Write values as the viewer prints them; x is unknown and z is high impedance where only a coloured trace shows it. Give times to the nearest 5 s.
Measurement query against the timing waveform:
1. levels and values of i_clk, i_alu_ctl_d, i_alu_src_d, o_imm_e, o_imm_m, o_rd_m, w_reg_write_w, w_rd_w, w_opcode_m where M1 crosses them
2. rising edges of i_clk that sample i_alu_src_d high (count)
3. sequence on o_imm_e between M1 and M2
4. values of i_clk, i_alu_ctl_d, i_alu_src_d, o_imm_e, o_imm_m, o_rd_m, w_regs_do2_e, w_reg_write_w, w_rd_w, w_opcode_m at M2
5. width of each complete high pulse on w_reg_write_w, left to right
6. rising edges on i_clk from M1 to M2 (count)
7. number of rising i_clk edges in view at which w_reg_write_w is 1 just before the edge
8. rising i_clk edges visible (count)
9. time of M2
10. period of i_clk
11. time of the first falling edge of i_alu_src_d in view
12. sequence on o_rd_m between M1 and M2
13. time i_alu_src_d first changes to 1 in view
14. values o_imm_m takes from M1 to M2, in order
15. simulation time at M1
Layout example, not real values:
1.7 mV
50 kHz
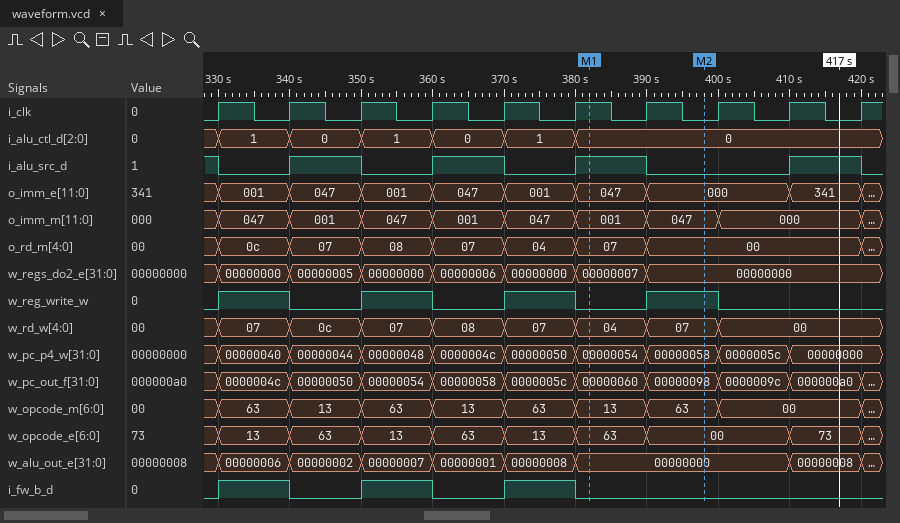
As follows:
i_clk=1, i_alu_ctl_d=0, i_alu_src_d=1, o_imm_e=047, o_imm_m=001, o_rd_m=07, w_reg_write_w=0, w_rd_w=04, w_opcode_m=13
5
047, 000
i_clk=0, i_alu_ctl_d=0, i_alu_src_d=0, o_imm_e=000, o_imm_m=047, o_rd_m=00, w_regs_do2_e=00000000, w_reg_write_w=1, w_rd_w=07, w_opcode_m=63
10 s, 10 s, 10 s, 10 s
1
4
10
400 s
10 s
330 s
07, 00
340 s
001, 047
380 s
